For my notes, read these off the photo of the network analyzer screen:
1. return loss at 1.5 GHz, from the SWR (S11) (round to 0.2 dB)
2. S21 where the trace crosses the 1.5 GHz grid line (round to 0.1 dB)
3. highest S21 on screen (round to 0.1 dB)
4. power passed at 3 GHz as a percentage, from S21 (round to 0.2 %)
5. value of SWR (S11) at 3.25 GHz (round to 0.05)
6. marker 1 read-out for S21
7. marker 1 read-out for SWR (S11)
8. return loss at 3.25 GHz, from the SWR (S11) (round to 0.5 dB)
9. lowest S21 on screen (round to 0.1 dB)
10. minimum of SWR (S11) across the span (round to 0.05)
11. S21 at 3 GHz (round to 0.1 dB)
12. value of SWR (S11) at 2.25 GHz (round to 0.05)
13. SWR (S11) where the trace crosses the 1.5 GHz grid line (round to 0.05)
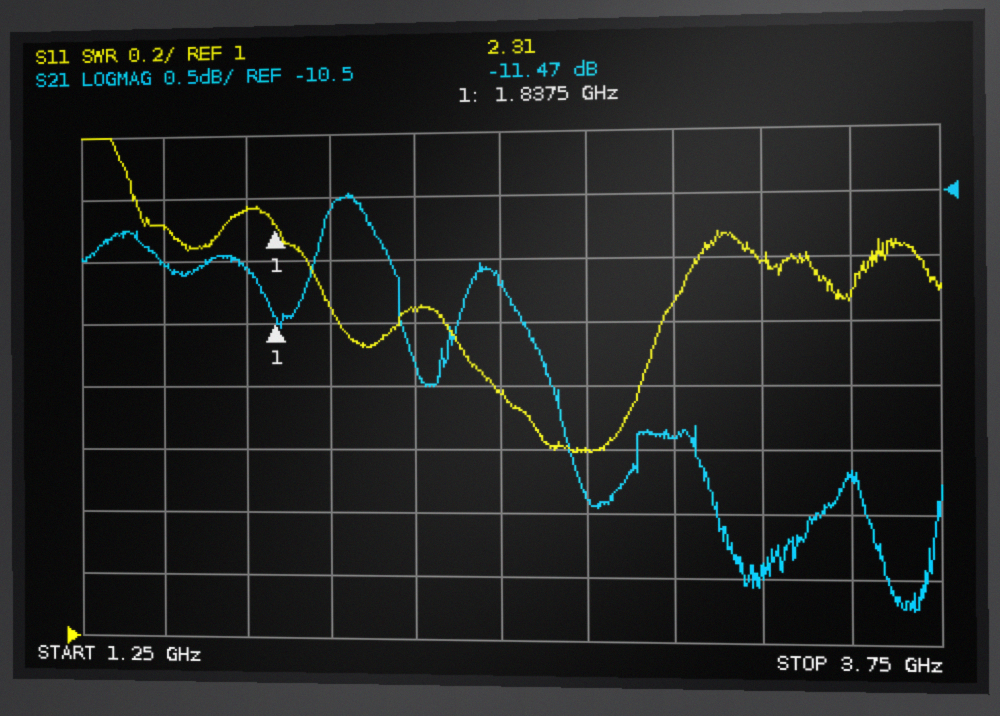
8.0 dB
-11.0 dB
-10.5 dB
5.8 %
2.20
-11.47 dB
2.31
8.5 dB
-13.7 dB
1.60
-12.4 dB
2.05
2.30
